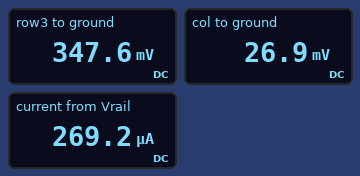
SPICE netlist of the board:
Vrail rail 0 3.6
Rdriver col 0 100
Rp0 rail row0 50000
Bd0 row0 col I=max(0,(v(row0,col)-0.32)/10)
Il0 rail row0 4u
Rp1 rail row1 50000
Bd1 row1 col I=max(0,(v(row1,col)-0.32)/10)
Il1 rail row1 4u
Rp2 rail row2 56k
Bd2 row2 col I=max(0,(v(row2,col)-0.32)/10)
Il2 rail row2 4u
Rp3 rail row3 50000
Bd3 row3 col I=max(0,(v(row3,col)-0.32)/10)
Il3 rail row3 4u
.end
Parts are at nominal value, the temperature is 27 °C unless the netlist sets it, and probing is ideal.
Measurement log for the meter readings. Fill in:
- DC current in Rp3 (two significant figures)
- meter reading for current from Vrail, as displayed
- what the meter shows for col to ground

65 µA
269.2 µA
26.9 mV
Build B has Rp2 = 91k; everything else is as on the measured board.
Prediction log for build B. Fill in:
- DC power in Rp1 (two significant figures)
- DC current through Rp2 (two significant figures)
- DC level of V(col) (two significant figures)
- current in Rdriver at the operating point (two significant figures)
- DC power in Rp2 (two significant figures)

210 µW
36 µA
25 mV
250 µA
120 µW
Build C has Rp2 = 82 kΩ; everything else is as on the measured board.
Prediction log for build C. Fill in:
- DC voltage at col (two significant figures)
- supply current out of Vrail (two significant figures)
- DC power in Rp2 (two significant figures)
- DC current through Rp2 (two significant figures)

25 mV
250 µA
130 µW
40 µA
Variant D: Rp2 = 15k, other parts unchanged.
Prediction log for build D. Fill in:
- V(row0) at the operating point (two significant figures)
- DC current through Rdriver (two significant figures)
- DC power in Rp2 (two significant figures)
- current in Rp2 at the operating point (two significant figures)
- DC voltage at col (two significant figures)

360 mV
430 µA
700 µW
220 µA
43 mV
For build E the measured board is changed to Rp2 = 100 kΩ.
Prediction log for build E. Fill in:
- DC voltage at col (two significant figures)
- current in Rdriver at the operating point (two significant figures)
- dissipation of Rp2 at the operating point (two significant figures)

24 mV
240 µA
110 µW
